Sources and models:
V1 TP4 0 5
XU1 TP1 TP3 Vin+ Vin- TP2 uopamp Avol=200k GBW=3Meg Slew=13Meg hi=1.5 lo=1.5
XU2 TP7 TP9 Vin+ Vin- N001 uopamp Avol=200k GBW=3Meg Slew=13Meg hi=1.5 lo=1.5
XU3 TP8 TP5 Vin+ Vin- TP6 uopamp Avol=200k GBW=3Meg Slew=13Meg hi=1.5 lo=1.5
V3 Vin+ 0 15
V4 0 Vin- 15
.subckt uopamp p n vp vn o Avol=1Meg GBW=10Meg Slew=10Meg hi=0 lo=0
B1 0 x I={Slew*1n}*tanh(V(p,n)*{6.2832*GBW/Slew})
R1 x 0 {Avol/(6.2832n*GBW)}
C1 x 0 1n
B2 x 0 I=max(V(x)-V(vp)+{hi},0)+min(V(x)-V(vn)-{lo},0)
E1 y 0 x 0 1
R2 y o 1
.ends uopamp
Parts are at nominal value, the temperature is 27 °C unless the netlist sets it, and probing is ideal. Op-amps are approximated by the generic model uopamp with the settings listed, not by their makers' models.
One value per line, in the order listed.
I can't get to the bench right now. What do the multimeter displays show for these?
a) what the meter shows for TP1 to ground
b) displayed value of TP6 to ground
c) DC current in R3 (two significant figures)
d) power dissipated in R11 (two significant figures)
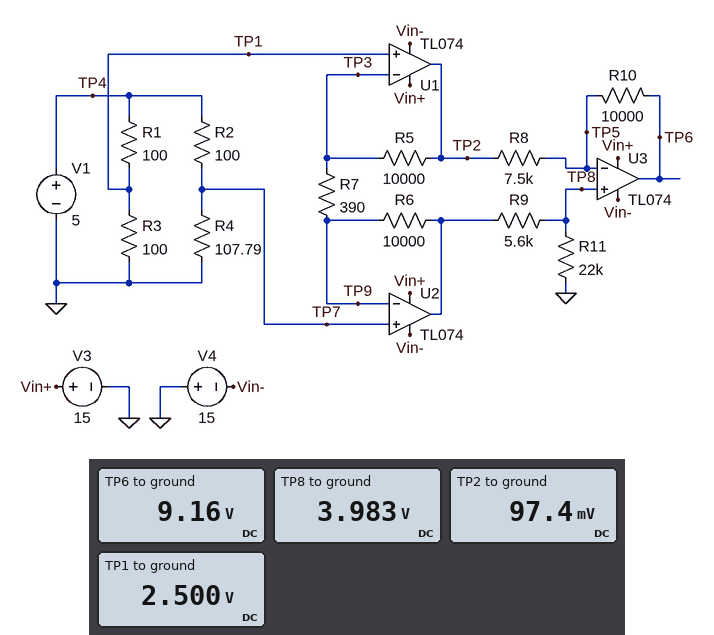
2.500 V
9.16 V
25 mA
720 µW
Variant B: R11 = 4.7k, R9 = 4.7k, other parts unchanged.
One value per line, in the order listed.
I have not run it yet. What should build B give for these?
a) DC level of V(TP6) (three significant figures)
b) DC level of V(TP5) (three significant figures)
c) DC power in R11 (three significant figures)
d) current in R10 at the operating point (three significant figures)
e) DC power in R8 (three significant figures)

5.70 V
2.50 V
1.33 mW
320 µA
768 µW
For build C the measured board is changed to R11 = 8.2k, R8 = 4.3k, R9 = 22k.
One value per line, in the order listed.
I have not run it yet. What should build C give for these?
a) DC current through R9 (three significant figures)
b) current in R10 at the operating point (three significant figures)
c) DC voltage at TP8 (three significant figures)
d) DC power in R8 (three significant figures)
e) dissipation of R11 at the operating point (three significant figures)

165 µA
293 µA
1.36 V
369 µW
224 µW
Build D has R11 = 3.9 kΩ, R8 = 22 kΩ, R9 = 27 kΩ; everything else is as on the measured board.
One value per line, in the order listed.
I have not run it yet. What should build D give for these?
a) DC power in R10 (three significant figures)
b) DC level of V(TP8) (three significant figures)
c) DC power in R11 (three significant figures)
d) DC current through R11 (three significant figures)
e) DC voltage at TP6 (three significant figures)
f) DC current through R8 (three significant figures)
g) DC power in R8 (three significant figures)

5.87 µW
631 mV
102 µW
162 µA
873 mV
24.2 µA
12.9 µW
